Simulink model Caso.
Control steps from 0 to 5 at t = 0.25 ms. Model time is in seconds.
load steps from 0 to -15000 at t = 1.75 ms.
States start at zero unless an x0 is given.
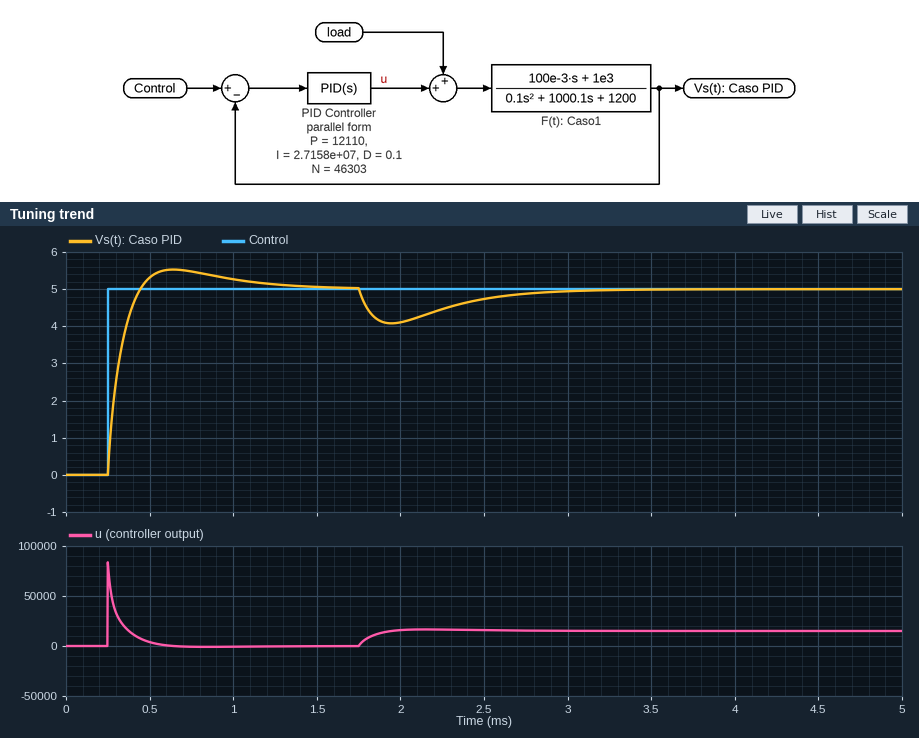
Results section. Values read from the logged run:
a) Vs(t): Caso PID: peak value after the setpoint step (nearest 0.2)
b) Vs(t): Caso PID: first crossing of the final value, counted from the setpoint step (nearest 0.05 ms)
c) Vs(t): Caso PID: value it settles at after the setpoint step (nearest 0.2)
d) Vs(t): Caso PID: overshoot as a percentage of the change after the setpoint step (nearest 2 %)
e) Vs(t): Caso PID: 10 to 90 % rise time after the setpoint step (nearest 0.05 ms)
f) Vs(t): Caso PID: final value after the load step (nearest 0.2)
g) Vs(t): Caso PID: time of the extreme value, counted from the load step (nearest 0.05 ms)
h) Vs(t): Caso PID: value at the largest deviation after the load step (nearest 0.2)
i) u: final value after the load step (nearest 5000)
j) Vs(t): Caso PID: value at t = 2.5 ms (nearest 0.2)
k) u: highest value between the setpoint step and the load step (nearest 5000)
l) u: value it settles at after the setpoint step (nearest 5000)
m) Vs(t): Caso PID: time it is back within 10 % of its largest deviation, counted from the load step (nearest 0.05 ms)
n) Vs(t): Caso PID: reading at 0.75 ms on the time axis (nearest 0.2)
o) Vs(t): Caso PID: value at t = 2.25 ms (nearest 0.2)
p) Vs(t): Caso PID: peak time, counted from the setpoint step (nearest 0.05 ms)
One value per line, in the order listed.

5.6
0.20 ms
5.0
10 %
0.15 ms
5.0
0.20 ms
4.0
15000
4.8
85000
0
1.10 ms
5.4
4.4
0.40 ms
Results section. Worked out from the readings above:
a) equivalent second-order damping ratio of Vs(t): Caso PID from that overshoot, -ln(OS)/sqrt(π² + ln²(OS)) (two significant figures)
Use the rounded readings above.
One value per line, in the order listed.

0.59
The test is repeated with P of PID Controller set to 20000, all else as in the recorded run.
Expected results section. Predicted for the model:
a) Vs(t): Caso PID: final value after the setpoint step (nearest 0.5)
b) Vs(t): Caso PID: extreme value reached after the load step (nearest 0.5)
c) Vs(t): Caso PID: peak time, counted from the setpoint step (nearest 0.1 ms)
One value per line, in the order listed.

5.0
4.5
0.3 ms
